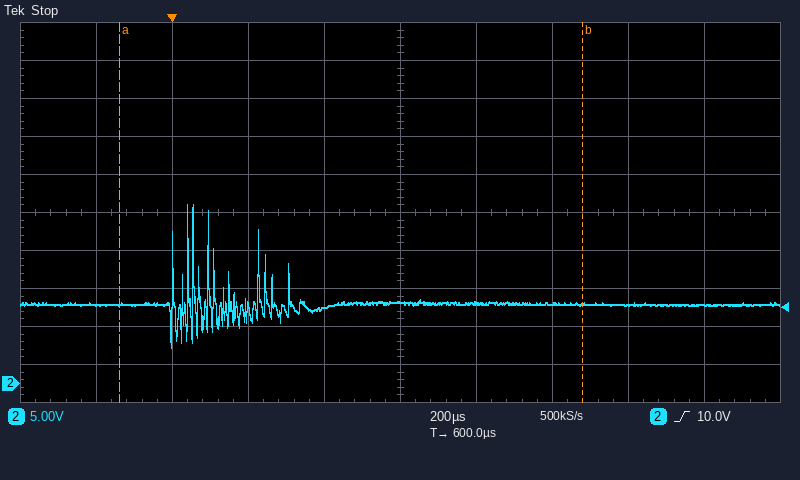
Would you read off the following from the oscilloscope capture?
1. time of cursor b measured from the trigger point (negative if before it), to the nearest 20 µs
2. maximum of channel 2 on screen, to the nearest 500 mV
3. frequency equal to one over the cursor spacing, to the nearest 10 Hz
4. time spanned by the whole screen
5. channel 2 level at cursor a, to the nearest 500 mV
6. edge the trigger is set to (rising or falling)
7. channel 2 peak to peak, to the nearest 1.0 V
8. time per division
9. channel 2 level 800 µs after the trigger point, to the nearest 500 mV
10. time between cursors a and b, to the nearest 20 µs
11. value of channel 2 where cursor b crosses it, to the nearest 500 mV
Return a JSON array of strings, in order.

["+1.08 ms", "23.5 V", "820 Hz", "2 ms", "10.5 V", "rising", "19.0 V", "200 µs", "10.5 V", "1.22 ms", "10.5 V"]
